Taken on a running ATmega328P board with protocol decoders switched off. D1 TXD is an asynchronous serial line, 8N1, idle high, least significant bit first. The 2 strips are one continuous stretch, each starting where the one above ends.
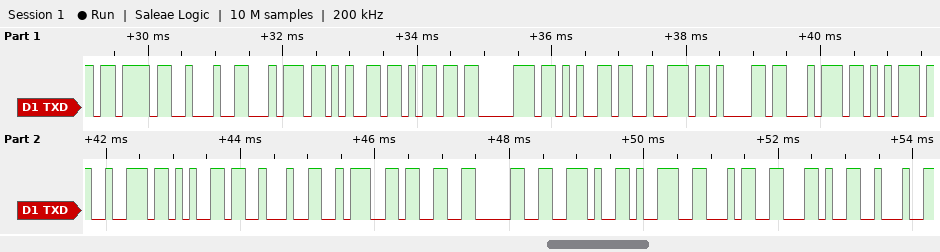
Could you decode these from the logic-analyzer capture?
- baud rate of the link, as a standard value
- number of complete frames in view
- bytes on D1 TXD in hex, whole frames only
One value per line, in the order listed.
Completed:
9600 baud
22
7B 22 74 65 6D 70 65 72 61 74 75 72 65 22 3A 33 30 2E 39 34 2C 22
